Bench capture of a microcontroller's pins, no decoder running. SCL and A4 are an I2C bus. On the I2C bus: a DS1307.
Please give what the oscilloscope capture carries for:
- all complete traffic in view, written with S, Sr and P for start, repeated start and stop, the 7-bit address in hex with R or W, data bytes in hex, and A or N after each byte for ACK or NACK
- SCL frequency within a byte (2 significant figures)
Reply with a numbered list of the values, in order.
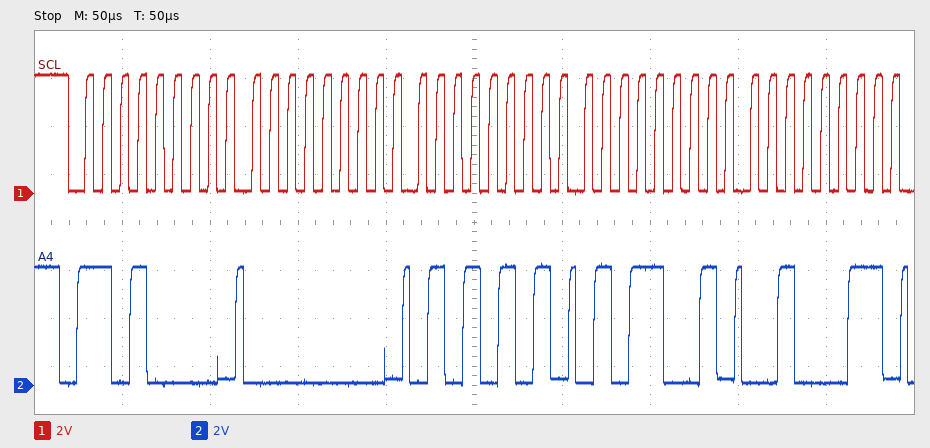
1. S 68W A 00 A 55 A 59 A 23 A
2. 100 kHz
